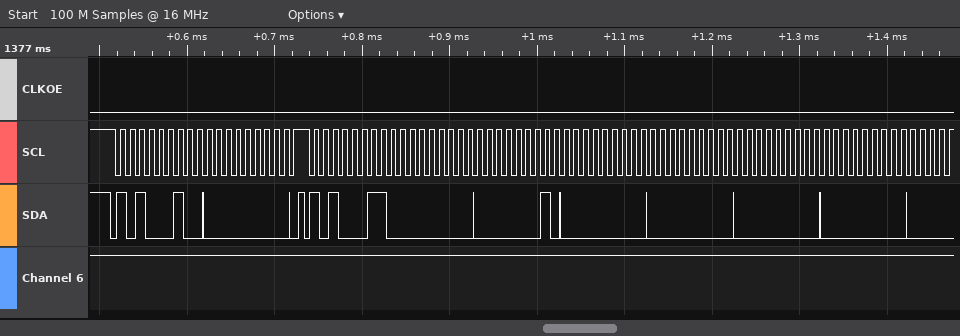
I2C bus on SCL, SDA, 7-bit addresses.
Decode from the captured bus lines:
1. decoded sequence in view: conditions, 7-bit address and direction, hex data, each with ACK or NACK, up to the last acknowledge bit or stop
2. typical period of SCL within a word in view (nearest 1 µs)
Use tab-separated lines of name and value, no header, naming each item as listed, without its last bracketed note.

decoded sequence in view: conditions, 7-bit address and direction, hex data, each with ACK or NACK, up to the last acknowledge bit or stop	start, address 51 write ACK, 00 ACK, stop, start, address 51 read ACK, 00 ACK, 02 ACK, 00 ACK, 00 ACK, 00 ACK, 00 ACK
typical period of SCL within a word in view	11 µs
